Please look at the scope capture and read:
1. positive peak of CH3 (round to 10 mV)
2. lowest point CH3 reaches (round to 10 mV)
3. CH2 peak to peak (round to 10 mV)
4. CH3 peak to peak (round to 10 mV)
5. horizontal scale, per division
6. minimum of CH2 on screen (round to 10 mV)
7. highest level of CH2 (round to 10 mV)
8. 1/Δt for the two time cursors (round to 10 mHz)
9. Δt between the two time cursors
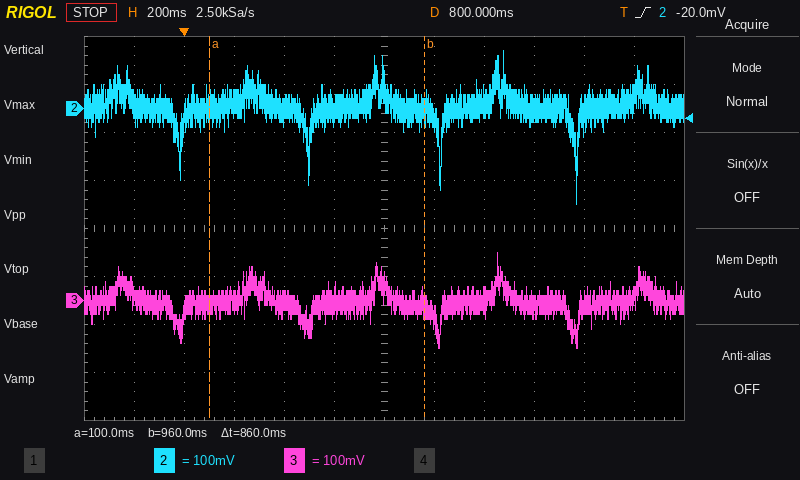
100 mV
-100 mV
320 mV
200 mV
200 ms
-200 mV
120 mV
1.16 Hz
860 ms
